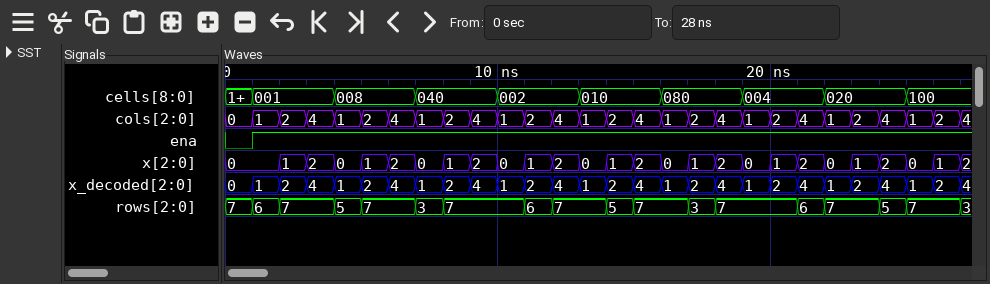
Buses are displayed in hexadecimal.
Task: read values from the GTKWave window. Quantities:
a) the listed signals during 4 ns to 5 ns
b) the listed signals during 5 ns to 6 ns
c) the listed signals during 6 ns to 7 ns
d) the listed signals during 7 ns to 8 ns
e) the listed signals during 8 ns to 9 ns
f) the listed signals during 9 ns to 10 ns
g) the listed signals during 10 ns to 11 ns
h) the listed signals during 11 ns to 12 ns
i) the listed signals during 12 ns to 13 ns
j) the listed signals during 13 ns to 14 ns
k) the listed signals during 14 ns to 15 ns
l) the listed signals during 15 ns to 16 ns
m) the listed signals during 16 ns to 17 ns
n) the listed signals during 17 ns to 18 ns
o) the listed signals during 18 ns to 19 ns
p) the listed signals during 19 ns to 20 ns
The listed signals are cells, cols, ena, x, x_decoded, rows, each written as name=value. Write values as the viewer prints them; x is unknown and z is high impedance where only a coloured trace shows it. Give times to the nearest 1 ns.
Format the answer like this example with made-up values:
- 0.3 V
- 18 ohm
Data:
- cells=008, cols=1, ena=1, x=0, x_decoded=1, rows=5
- cells=008, cols=2, ena=1, x=1, x_decoded=2, rows=7
- cells=008, cols=4, ena=1, x=2, x_decoded=4, rows=7
- cells=040, cols=1, ena=1, x=0, x_decoded=1, rows=3
- cells=040, cols=2, ena=1, x=1, x_decoded=2, rows=7
- cells=040, cols=4, ena=1, x=2, x_decoded=4, rows=7
- cells=002, cols=1, ena=1, x=0, x_decoded=1, rows=7
- cells=002, cols=2, ena=1, x=1, x_decoded=2, rows=6
- cells=002, cols=4, ena=1, x=2, x_decoded=4, rows=7
- cells=010, cols=1, ena=1, x=0, x_decoded=1, rows=7
- cells=010, cols=2, ena=1, x=1, x_decoded=2, rows=5
- cells=010, cols=4, ena=1, x=2, x_decoded=4, rows=7
- cells=080, cols=1, ena=1, x=0, x_decoded=1, rows=7
- cells=080, cols=2, ena=1, x=1, x_decoded=2, rows=3
- cells=080, cols=4, ena=1, x=2, x_decoded=4, rows=7
- cells=004, cols=1, ena=1, x=0, x_decoded=1, rows=7
